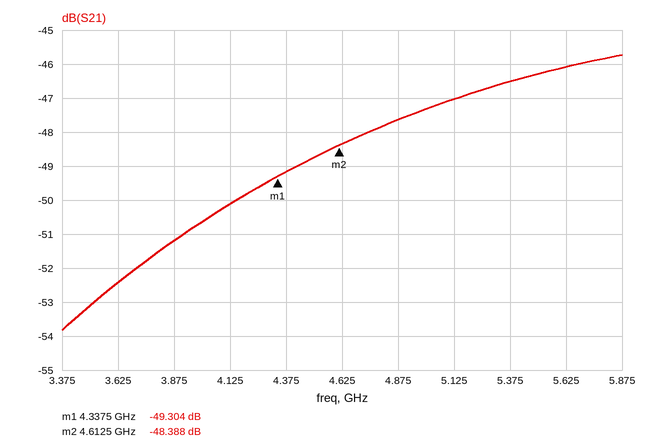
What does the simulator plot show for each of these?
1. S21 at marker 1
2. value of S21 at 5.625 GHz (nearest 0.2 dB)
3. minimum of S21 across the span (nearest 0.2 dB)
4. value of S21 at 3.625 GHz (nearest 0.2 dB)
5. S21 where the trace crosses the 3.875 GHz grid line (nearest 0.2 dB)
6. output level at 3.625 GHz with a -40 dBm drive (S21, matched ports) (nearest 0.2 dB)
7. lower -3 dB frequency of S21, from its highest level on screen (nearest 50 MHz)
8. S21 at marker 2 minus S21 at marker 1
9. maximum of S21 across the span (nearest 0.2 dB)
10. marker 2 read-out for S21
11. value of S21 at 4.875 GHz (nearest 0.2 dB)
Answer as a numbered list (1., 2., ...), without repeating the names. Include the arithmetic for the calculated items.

1. -49.304 dB
2. -46.0 dB
3. -53.8 dB
4. -52.4 dB
5. -51.2 dB
6. -40 dBm + (-52.4 dB) = -92.4 dBm
7. 4.50 GHz
8. -48.388 − (-49.304) = 0.916 dB
9. -45.8 dB
10. -48.388 dB
11. -47.6 dB
